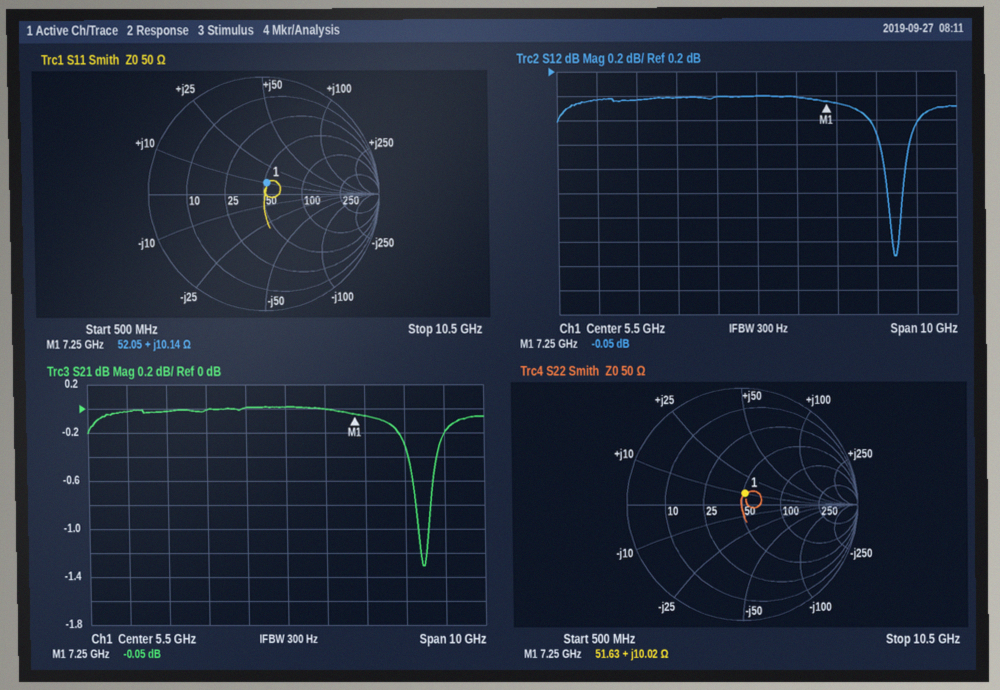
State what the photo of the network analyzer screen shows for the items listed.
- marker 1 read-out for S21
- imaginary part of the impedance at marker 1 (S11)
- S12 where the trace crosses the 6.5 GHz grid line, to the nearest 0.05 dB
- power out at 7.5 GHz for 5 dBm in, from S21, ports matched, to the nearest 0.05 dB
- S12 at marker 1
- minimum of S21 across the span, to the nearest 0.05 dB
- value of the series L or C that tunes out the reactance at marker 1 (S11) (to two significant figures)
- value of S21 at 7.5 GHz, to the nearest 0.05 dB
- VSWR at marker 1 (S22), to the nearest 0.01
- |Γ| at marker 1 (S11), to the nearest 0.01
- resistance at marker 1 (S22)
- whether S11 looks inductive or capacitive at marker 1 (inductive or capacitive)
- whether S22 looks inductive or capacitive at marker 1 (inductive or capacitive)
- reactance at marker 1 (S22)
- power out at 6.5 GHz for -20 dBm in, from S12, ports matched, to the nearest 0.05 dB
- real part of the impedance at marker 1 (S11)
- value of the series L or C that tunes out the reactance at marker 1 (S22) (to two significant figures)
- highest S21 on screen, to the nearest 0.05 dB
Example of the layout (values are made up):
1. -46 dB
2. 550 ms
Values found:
1. -0.05 dB
2. +10.14 Ω
3. 0.00 dB
4. 4.95 dBm
5. -0.05 dB
6. -1.30 dB
7. 2.2 pF
8. -0.05 dB
9. 1.22
10. 0.10
11. 51.63 Ω
12. inductive
13. inductive
14. +10.02 Ω
15. -20.00 dBm
16. 52.05 Ω
17. 2.2 pF
18. 0.00 dB
